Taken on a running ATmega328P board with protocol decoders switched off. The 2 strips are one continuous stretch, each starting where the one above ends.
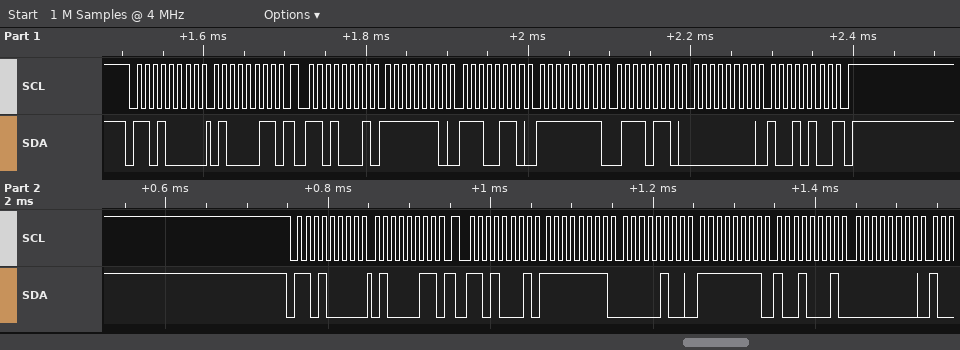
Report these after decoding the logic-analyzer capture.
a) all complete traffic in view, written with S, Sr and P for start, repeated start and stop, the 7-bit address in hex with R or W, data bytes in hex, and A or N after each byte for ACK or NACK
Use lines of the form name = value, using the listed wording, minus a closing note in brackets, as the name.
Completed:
all complete traffic in view, written with S, Sr and P for start, repeated start and stop, the 7-bit address in hex with R or W, data bytes in hex, and A or N after each byte for ACK or NACK = S 68W A 43 A Sr 68R A FE A E6 A FF A 76 A 00 A 94 N P S 68W A 43 A Sr 68R A FF A 04 A FF A 91 A 00 A
